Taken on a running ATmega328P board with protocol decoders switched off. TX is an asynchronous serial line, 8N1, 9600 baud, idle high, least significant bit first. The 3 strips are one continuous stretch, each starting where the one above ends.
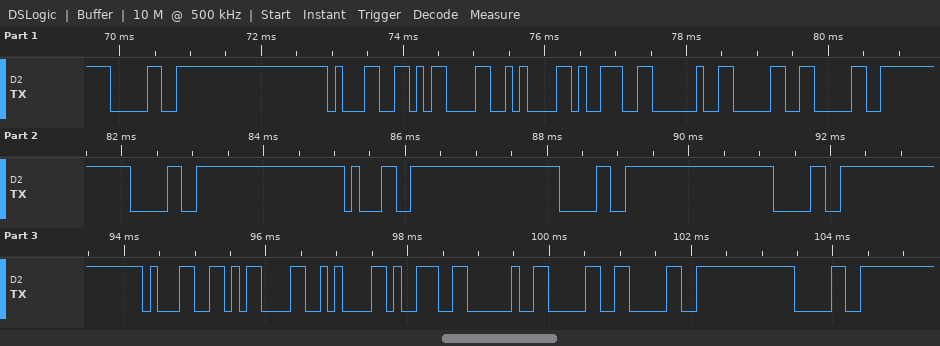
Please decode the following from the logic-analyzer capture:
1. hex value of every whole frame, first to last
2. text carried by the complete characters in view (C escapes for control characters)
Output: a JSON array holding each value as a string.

["30 31 0D 0A 39 20 30 30 30 31 30 30 31 0D 0A 39 20 30 30 30", "\"01\\r\\n9 0001001\\r\\n9 000\""]
